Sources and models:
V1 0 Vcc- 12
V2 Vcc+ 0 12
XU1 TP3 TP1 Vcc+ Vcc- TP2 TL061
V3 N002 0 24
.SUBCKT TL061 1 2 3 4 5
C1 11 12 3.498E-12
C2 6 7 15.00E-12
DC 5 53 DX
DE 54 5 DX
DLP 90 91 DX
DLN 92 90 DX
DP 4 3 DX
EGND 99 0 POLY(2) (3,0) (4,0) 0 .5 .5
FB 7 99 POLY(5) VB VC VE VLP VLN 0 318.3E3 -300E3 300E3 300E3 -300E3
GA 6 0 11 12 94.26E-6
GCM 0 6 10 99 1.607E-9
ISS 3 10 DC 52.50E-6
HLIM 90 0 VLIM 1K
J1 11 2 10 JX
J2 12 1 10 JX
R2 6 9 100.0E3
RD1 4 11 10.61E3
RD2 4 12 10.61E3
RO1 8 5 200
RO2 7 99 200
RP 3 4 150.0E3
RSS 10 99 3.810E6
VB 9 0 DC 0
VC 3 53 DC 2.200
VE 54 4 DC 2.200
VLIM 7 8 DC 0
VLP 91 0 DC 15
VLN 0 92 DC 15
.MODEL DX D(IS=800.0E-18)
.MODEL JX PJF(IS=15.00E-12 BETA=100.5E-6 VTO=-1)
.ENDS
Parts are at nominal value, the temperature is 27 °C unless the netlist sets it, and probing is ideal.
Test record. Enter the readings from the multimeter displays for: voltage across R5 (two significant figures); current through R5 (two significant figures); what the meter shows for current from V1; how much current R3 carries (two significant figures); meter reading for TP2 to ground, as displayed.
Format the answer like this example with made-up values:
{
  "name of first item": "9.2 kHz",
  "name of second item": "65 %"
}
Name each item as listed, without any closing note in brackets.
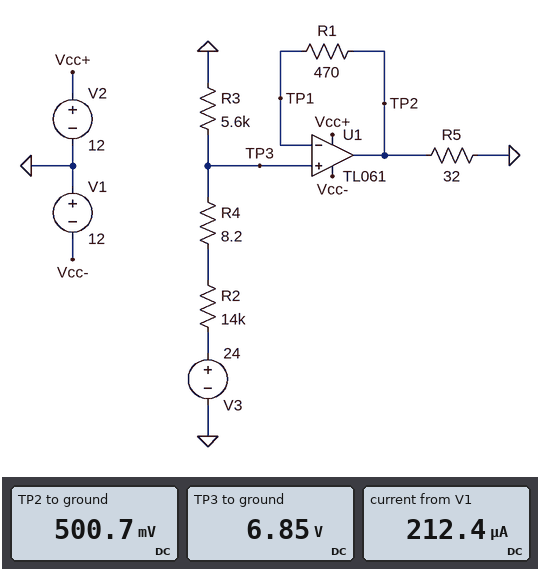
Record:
{
  "voltage across R5": "500 mV",
  "current through R5": "16 mA",
  "what the meter shows for current from V1": "212.4 µA",
  "how much current R3 carries": "1.2 mA",
  "meter reading for TP2 to ground, as displayed": "500.7 mV"
}
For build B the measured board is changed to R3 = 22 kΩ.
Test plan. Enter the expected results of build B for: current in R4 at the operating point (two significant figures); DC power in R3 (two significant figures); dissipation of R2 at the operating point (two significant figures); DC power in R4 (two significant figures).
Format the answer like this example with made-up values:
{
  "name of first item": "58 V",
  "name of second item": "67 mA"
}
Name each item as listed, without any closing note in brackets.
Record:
{
  "current in R4 at the operating point": "670 µA",
  "DC power in R3": "9.8 mW",
  "dissipation of R2 at the operating point": "6.2 mW",
  "DC power in R4": "3.6 µW"
}
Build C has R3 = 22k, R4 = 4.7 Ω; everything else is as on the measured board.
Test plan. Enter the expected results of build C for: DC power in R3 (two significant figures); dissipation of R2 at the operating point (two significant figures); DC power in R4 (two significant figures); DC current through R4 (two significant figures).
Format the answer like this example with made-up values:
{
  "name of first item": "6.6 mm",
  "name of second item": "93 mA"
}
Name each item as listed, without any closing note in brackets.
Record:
{
  "DC power in R3": "9.8 mW",
  "dissipation of R2 at the operating point": "6.2 mW",
  "DC power in R4": "2.1 µW",
  "DC current through R4": "670 µA"
}
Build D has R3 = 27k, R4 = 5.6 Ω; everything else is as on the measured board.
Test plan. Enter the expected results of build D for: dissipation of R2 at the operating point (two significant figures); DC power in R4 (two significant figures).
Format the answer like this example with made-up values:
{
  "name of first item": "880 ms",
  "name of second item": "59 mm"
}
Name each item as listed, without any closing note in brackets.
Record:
{
  "dissipation of R2 at the operating point": "4.8 mW",
  "DC power in R4": "1.9 µW"
}
